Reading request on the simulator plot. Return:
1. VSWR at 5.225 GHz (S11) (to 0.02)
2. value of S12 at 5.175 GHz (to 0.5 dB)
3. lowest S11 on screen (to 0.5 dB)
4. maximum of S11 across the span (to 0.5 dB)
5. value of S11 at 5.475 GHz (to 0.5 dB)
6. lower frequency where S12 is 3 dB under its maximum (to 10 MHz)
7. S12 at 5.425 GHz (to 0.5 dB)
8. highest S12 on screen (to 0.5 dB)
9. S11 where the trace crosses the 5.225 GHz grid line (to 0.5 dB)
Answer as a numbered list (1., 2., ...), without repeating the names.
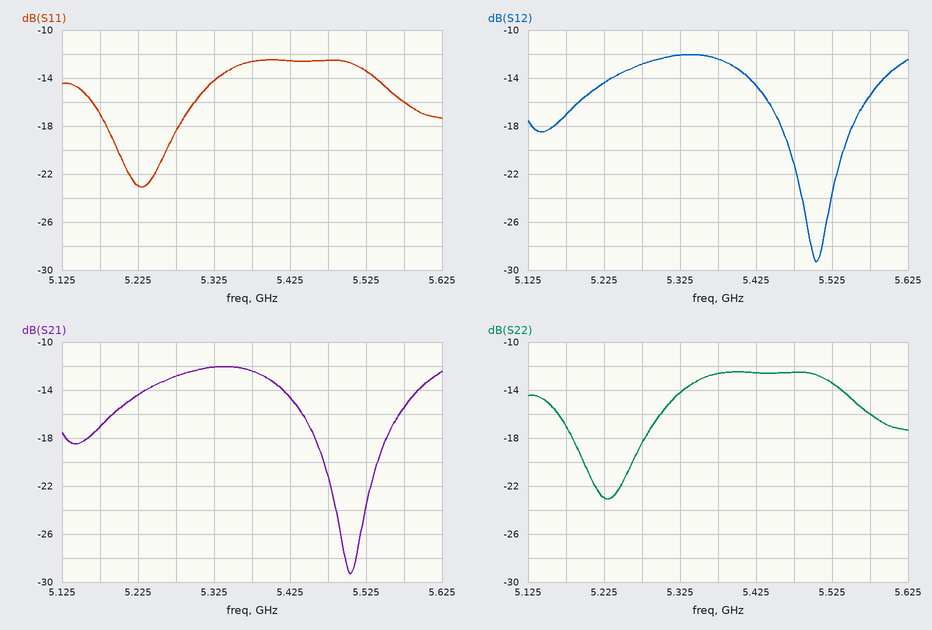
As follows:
1. 1.16
2. -17.0 dB
3. -23.0 dB
4. -12.5 dB
5. -12.5 dB
6. 5.21 GHz
7. -14.5 dB
8. -12.0 dB
9. -23.0 dB
